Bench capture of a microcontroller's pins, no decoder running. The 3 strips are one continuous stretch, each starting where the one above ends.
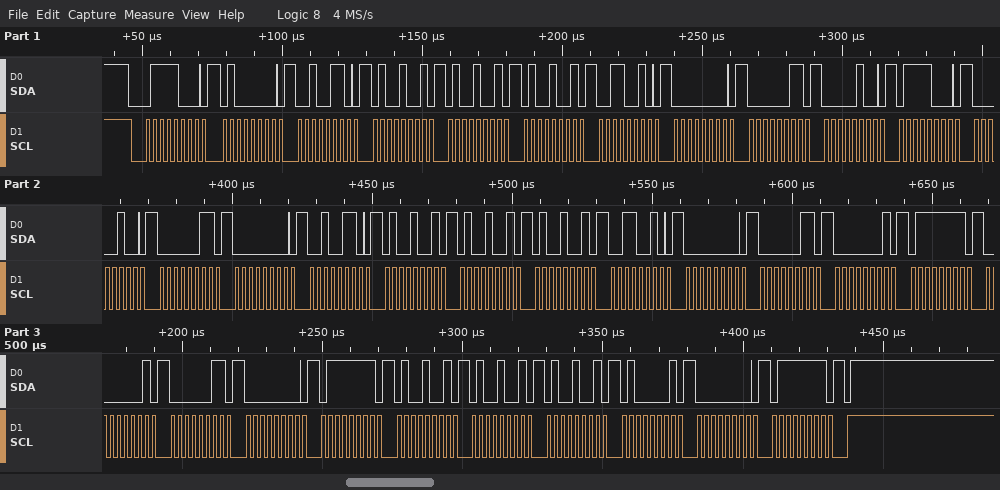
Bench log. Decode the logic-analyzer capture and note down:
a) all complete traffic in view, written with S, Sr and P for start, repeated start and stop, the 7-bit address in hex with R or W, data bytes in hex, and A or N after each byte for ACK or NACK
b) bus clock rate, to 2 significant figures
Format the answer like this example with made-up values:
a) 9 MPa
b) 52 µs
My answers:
a) S 3CW A 40 A 26 A 49 A 49 A 49 A 32 A 00 A 03 A 04 A 78 A 04 A 03 A 00 A 26 A 49 A 49 A 49 A 32 A 00 A 03 A 01 A 7F A 01 A 03 A 00 A 7F A 49 A 49 A 49 A 41 A 00 A 7F A P
b) 400 kHz
